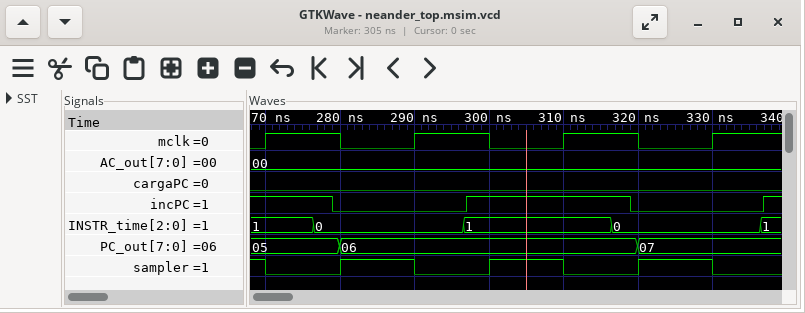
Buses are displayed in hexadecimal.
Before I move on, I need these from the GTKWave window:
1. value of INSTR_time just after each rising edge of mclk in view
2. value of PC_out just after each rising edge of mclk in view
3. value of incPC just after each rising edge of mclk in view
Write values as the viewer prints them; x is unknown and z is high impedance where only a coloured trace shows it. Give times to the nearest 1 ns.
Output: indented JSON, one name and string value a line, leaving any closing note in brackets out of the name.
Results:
{
  "value of INSTR_time just after each rising edge of mclk in view": "1, 0, 1, 0",
  "value of PC_out just after each rising edge of mclk in view": "05, 06, 06, 07",
  "value of incPC just after each rising edge of mclk in view": "1 0 1 0"
}
